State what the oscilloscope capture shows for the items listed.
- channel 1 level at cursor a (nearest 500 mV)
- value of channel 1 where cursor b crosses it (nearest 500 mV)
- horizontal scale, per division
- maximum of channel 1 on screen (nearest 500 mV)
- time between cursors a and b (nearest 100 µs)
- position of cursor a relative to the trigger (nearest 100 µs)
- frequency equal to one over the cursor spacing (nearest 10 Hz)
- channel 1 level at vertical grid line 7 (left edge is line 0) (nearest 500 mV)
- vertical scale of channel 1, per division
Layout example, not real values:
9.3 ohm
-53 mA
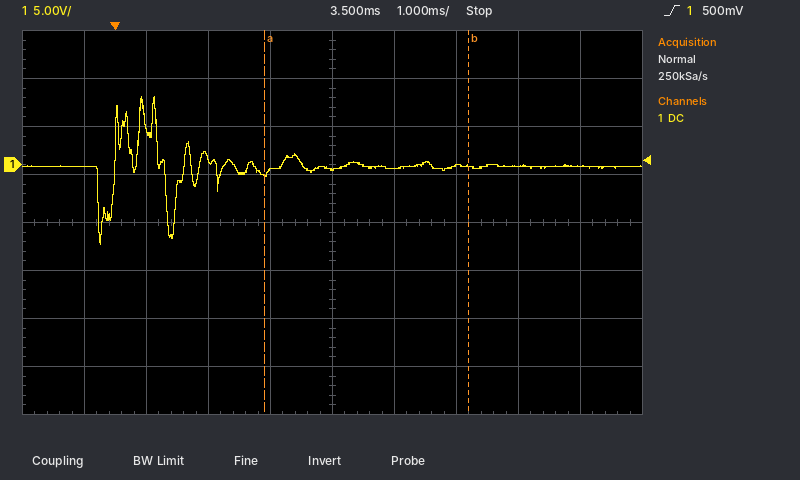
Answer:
-1.0 V
0.0 V
1 ms
7.0 V
3.3 ms
+2.4 ms
300 Hz
0.0 V
5 V
